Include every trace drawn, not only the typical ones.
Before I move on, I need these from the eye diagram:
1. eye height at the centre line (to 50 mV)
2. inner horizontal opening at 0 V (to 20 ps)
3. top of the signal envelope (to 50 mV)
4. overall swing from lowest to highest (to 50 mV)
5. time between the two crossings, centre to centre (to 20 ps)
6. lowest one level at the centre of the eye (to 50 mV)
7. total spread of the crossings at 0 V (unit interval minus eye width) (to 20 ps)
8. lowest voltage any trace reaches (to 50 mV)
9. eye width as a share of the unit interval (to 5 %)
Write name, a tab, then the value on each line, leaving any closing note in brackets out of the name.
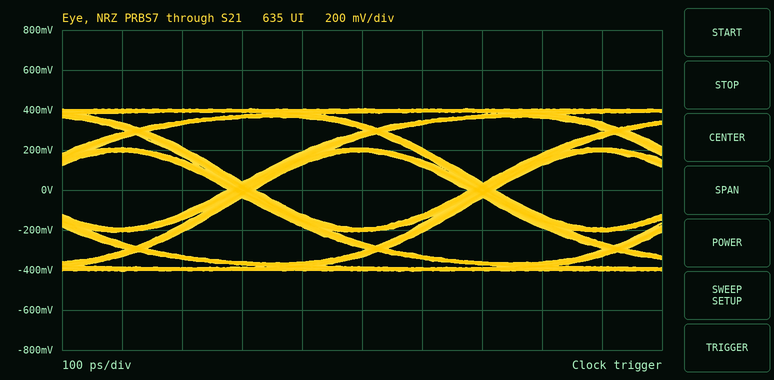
eye height at the centre line	400 mV
inner horizontal opening at 0 V	360 ps
top of the signal envelope	400 mV
overall swing from lowest to highest	800 mV
time between the two crossings, centre to centre	400 ps
lowest one level at the centre of the eye	200 mV
total spread of the crossings at 0 V (unit interval minus eye width)	40 ps
lowest voltage any trace reaches	-400 mV
eye width as a share of the unit interval	90 %
